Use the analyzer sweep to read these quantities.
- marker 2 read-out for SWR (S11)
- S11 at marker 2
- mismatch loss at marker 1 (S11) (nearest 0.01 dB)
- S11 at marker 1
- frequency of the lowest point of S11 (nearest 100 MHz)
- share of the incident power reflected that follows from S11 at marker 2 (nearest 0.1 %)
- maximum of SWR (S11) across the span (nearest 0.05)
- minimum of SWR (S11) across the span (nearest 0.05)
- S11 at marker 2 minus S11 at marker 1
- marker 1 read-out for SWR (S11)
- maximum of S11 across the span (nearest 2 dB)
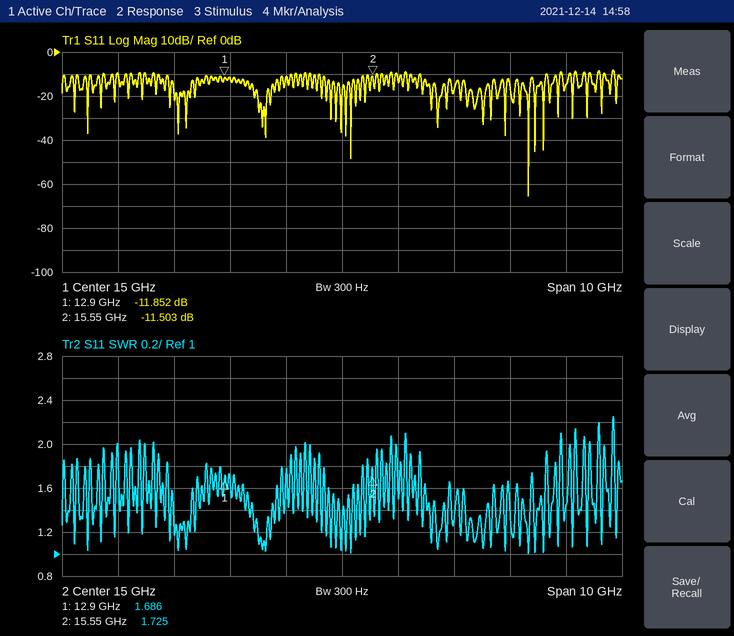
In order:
1.725
-11.503 dB
0.29 dB
-11.852 dB
18.3 GHz
7.1 %
2.25
1.00
0.349 dB
1.686
-8 dB
